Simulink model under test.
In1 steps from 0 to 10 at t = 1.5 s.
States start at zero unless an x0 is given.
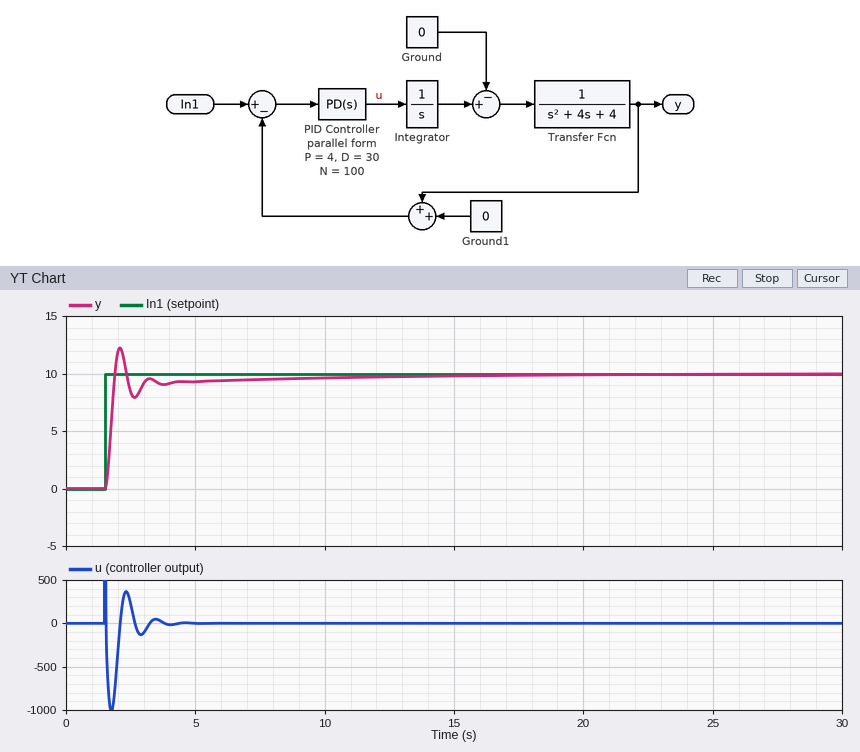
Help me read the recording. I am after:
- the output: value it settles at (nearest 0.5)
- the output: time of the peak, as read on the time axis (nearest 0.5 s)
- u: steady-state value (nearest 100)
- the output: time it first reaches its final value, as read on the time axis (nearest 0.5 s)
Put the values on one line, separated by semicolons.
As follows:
10.0; 2.0 s; 0; 2.0 s
